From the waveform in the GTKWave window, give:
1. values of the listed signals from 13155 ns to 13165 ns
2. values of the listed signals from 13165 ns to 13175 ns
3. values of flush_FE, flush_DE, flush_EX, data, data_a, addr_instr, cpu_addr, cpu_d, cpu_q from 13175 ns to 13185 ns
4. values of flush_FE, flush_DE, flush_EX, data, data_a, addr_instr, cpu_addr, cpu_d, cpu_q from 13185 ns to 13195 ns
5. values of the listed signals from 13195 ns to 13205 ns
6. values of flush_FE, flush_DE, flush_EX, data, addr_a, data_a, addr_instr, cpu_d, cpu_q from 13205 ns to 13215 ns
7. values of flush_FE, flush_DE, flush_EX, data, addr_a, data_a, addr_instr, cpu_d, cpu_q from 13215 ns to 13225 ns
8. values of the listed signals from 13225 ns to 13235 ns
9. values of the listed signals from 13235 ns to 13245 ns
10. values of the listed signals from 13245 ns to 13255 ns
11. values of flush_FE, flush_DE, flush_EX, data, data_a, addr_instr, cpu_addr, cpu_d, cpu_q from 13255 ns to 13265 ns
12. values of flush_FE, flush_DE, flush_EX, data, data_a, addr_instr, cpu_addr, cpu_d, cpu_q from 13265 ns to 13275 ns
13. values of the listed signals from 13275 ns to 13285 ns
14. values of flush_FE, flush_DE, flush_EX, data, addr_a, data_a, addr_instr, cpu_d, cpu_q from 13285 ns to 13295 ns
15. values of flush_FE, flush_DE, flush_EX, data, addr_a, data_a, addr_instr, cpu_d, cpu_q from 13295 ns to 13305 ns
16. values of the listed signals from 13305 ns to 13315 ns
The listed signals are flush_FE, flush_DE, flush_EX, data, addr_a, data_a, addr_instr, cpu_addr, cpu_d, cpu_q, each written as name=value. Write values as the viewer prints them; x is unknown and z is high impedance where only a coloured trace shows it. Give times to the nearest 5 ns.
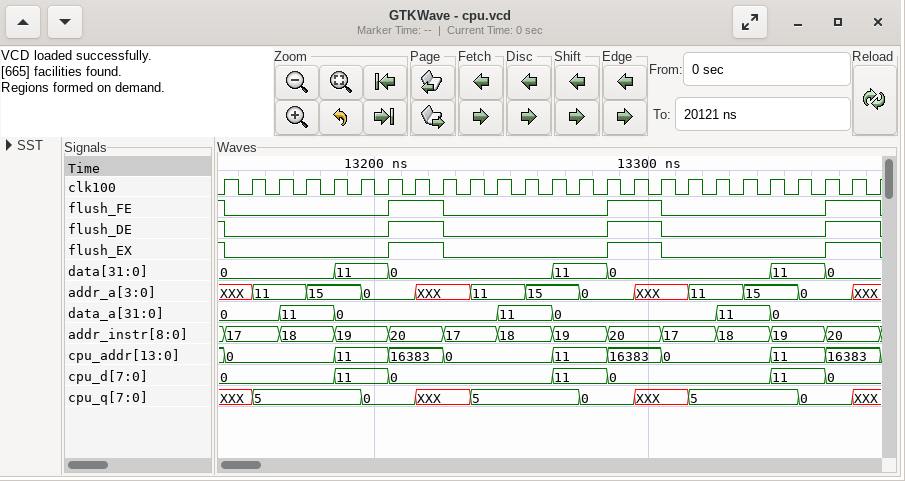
flush_FE=0, flush_DE=0, flush_EX=0, data=0, addr_a=11, data_a=0, addr_instr=17, cpu_addr=0, cpu_d=0, cpu_q=5
flush_FE=0, flush_DE=0, flush_EX=0, data=0, addr_a=11, data_a=11, addr_instr=18, cpu_addr=0, cpu_d=0, cpu_q=5
flush_FE=0, flush_DE=0, flush_EX=0, data=0, data_a=11, addr_instr=18, cpu_addr=0, cpu_d=0, cpu_q=5
flush_FE=0, flush_DE=0, flush_EX=0, data=11, data_a=0, addr_instr=19, cpu_addr=11, cpu_d=11, cpu_q=5
flush_FE=0, flush_DE=0, flush_EX=0, data=11, addr_a=0, data_a=0, addr_instr=19, cpu_addr=11, cpu_d=11, cpu_q=0
flush_FE=1, flush_DE=1, flush_EX=1, data=0, addr_a=0, data_a=0, addr_instr=20, cpu_d=0, cpu_q=0
flush_FE=1, flush_DE=1, flush_EX=1, data=0, addr_a=XXX, data_a=0, addr_instr=20, cpu_d=0, cpu_q=XXX
flush_FE=0, flush_DE=0, flush_EX=0, data=0, addr_a=XXX, data_a=0, addr_instr=17, cpu_addr=0, cpu_d=0, cpu_q=XXX
flush_FE=0, flush_DE=0, flush_EX=0, data=0, addr_a=11, data_a=0, addr_instr=17, cpu_addr=0, cpu_d=0, cpu_q=5
flush_FE=0, flush_DE=0, flush_EX=0, data=0, addr_a=11, data_a=11, addr_instr=18, cpu_addr=0, cpu_d=0, cpu_q=5
flush_FE=0, flush_DE=0, flush_EX=0, data=0, data_a=11, addr_instr=18, cpu_addr=0, cpu_d=0, cpu_q=5
flush_FE=0, flush_DE=0, flush_EX=0, data=11, data_a=0, addr_instr=19, cpu_addr=11, cpu_d=11, cpu_q=5
flush_FE=0, flush_DE=0, flush_EX=0, data=11, addr_a=0, data_a=0, addr_instr=19, cpu_addr=11, cpu_d=11, cpu_q=0
flush_FE=1, flush_DE=1, flush_EX=1, data=0, addr_a=0, data_a=0, addr_instr=20, cpu_d=0, cpu_q=0
flush_FE=1, flush_DE=1, flush_EX=1, data=0, addr_a=XXX, data_a=0, addr_instr=20, cpu_d=0, cpu_q=XXX
flush_FE=0, flush_DE=0, flush_EX=0, data=0, addr_a=XXX, data_a=0, addr_instr=17, cpu_addr=0, cpu_d=0, cpu_q=XXX
